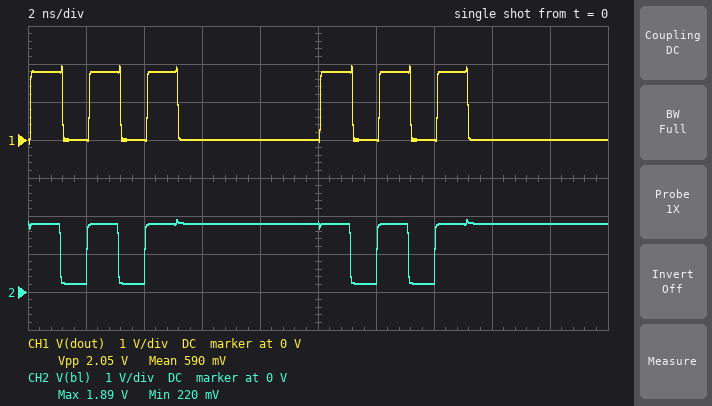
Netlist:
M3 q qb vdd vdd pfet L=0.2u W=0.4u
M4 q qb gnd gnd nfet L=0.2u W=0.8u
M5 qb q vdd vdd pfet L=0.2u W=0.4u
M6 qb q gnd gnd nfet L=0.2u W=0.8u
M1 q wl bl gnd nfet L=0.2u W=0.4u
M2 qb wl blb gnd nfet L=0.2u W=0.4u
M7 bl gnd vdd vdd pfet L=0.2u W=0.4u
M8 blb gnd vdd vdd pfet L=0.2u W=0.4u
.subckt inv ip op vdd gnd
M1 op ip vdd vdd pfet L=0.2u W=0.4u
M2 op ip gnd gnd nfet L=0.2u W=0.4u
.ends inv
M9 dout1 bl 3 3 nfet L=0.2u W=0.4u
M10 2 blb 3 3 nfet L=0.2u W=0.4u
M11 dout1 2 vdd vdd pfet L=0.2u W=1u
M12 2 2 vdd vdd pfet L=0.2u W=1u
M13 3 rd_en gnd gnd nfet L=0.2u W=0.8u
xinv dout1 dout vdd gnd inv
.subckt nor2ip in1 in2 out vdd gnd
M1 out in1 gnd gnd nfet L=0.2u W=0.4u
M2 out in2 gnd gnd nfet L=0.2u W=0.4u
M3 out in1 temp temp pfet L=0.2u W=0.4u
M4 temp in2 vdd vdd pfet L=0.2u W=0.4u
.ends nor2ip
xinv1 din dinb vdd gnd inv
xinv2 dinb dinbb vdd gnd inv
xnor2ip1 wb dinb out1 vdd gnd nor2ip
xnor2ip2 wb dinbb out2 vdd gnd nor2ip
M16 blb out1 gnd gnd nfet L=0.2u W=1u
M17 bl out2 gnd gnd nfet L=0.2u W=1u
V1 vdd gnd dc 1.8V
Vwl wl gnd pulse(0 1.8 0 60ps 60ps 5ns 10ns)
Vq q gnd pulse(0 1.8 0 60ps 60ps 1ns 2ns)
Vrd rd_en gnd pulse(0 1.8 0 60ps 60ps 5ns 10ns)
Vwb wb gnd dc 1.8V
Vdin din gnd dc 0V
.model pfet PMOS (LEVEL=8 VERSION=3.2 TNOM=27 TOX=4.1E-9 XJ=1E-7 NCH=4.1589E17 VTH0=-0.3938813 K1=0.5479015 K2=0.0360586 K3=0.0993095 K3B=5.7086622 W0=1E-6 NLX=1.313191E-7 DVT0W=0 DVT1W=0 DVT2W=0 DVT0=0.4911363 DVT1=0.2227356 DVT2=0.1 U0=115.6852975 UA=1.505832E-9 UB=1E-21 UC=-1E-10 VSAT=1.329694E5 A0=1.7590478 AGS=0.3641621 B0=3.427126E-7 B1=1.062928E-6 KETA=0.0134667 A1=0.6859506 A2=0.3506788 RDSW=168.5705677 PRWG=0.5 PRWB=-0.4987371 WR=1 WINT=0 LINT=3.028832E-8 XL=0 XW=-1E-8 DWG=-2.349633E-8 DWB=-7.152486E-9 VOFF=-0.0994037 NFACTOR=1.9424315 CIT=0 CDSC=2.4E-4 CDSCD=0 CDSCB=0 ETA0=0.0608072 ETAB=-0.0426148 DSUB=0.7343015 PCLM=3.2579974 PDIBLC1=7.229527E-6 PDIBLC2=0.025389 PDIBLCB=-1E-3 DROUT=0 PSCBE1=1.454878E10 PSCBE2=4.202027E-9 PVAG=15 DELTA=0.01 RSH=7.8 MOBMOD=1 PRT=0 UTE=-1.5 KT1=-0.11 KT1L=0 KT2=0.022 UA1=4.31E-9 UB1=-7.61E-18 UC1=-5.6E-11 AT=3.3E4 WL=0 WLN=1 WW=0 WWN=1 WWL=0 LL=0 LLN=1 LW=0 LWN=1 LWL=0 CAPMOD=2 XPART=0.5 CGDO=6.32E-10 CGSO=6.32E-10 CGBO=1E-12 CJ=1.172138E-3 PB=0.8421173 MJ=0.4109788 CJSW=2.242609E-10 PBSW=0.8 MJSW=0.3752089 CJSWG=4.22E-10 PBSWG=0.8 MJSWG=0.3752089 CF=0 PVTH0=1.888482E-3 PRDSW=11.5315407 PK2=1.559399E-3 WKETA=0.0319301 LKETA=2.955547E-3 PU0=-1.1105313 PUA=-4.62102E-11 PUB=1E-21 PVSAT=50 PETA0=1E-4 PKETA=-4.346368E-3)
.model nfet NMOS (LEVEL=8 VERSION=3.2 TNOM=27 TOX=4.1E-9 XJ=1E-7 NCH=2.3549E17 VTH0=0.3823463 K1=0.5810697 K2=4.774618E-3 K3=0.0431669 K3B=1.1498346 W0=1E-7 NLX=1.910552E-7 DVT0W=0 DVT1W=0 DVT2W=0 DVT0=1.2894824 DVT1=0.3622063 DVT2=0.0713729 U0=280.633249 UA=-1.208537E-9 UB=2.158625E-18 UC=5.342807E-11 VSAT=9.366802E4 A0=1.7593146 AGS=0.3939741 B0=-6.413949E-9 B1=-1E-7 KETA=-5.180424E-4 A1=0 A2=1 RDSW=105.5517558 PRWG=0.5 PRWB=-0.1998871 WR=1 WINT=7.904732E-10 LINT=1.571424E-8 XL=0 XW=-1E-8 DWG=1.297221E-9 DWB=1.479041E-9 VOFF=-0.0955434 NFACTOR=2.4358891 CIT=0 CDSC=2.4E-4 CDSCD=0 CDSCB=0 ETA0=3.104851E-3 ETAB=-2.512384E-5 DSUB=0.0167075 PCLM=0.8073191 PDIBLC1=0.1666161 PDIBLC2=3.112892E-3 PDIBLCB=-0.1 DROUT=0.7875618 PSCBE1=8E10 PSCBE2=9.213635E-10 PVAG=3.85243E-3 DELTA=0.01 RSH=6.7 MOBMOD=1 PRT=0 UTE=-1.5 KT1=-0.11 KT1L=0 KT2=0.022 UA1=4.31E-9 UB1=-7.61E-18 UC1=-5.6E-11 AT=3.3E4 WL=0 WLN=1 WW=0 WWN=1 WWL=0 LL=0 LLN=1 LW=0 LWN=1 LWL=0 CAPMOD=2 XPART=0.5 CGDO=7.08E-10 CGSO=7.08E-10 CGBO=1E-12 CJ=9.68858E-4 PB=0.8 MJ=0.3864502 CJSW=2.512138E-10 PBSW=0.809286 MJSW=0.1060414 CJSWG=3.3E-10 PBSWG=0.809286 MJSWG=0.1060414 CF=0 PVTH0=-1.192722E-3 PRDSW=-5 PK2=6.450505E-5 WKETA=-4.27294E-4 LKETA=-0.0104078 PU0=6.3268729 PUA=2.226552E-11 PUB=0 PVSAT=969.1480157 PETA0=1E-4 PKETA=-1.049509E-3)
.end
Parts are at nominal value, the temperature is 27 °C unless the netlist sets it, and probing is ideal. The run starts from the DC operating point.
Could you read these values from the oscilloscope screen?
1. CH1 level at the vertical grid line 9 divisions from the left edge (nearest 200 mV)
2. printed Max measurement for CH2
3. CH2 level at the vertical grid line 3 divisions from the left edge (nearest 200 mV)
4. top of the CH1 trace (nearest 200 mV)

0 V
1.89 V
1.8 V
2.0 V
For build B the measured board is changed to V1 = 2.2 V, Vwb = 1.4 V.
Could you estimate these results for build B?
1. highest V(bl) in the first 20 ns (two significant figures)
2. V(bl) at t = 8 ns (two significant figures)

2.3 V
2.2 V
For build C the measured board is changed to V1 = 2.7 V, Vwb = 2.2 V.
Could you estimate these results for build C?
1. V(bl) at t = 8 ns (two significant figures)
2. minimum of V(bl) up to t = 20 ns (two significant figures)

2.7 V
1.2 V
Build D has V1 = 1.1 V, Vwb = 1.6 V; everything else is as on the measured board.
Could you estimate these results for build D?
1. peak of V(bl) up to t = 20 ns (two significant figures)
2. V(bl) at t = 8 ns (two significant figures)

1.2 V
1.1 V
